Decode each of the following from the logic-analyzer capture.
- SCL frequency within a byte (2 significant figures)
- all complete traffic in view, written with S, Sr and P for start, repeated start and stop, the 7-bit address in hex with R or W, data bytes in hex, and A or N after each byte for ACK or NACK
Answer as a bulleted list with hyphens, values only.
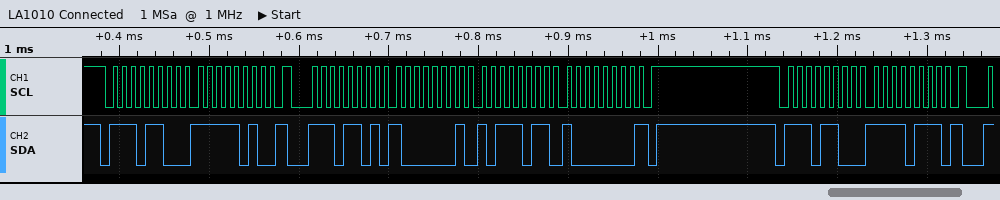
- 100 kHz
- S 76W A FA A Sr 76R A 81 A BB A 80 N P S 76W A F7 A
